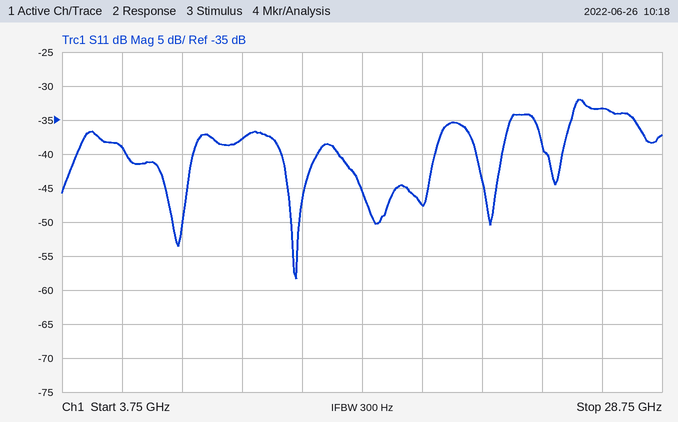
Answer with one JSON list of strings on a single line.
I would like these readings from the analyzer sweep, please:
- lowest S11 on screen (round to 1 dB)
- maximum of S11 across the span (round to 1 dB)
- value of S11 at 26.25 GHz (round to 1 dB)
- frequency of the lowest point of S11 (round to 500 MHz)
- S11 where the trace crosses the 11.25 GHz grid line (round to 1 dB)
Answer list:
["-58 dB", "-32 dB", "-33 dB", "13.5 GHz", "-38 dB"]
